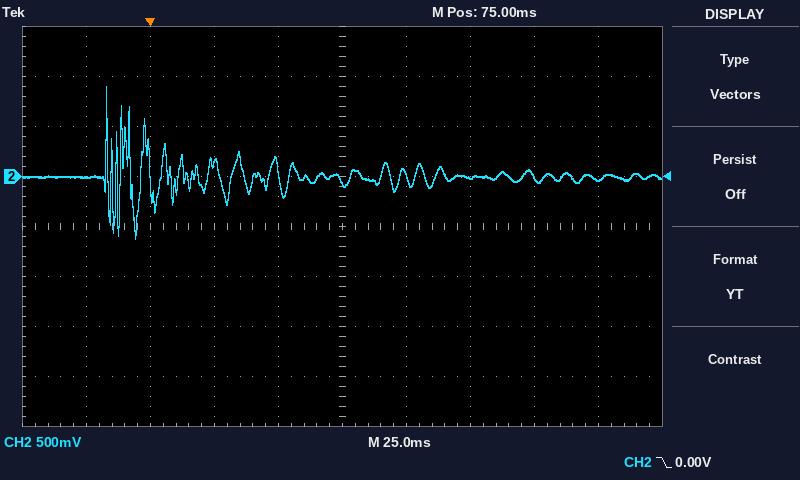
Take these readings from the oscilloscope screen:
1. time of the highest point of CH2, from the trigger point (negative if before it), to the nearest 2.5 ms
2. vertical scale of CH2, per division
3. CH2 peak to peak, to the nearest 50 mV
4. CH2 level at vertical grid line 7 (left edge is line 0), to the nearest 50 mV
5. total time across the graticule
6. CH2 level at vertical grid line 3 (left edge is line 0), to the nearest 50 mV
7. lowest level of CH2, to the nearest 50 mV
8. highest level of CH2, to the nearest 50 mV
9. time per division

-17.5 ms
500 mV
1.50 V
0 mV
250 ms
150 mV
-600 mV
900 mV
25 ms
